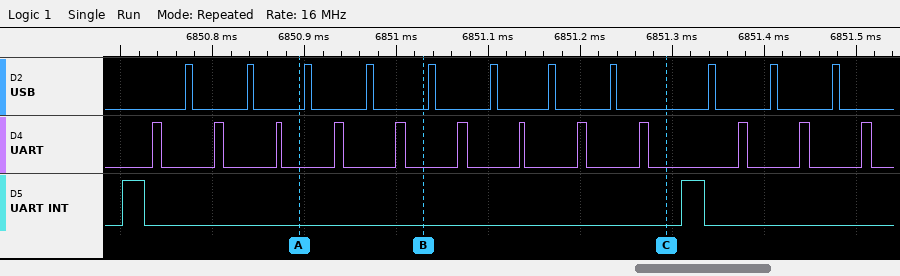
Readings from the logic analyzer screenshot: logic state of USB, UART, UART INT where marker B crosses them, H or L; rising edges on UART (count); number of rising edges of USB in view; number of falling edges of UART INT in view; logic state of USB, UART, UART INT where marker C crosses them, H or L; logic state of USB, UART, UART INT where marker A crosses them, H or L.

USB=L, UART=L, UART INT=L
12
11
2
USB=L, UART=L, UART INT=L
USB=L, UART=L, UART INT=L
